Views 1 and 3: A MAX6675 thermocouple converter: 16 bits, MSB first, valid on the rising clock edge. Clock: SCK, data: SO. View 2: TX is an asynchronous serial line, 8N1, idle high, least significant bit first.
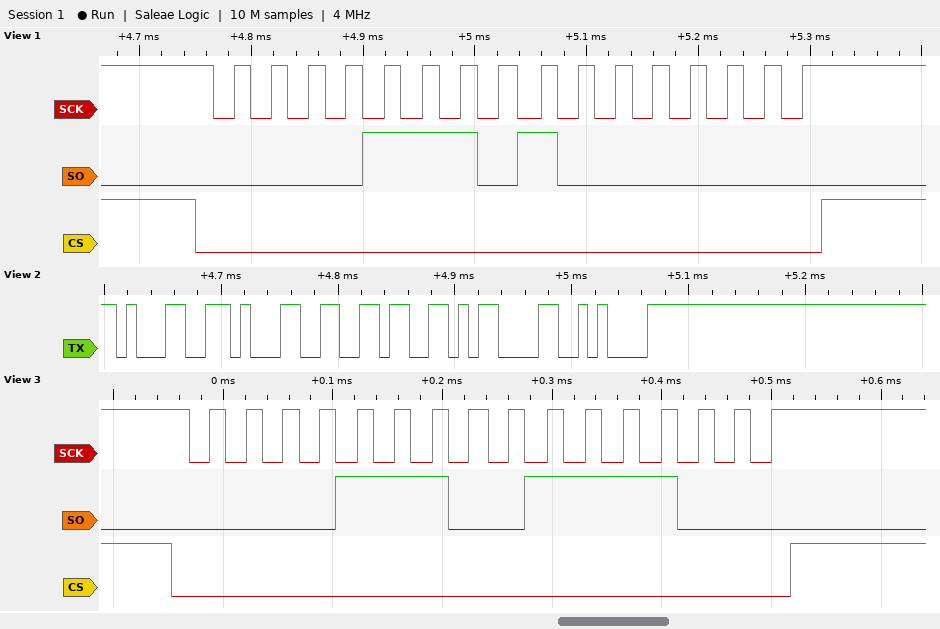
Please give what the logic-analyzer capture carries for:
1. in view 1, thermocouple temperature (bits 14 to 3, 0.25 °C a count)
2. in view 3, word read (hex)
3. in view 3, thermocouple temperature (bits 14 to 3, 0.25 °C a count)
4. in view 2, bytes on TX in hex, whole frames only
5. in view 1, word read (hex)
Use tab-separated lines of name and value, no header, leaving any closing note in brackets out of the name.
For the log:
in view 1, thermocouple temperature	116.00 °C
in view 3, word read	0x0E78
in view 3, thermocouple temperature	115.75 °C
in view 2, bytes on TX in hex, whole frames only	31 31 36 0D 0A
in view 1, word read	0x0E80
